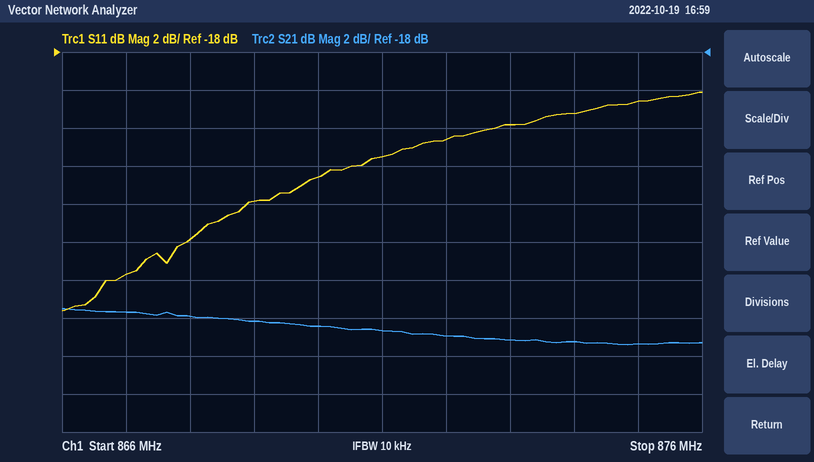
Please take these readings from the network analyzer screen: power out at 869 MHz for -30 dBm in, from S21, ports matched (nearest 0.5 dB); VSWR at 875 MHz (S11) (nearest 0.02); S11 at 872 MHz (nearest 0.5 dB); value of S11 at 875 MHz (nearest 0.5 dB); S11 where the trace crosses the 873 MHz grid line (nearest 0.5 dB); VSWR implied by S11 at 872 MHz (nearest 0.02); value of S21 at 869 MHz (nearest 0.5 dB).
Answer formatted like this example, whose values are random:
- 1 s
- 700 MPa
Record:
- -62.0 dBm
- 1.20
- -22.5 dB
- -20.5 dB
- -22.0 dB
- 1.16
- -32.0 dB
